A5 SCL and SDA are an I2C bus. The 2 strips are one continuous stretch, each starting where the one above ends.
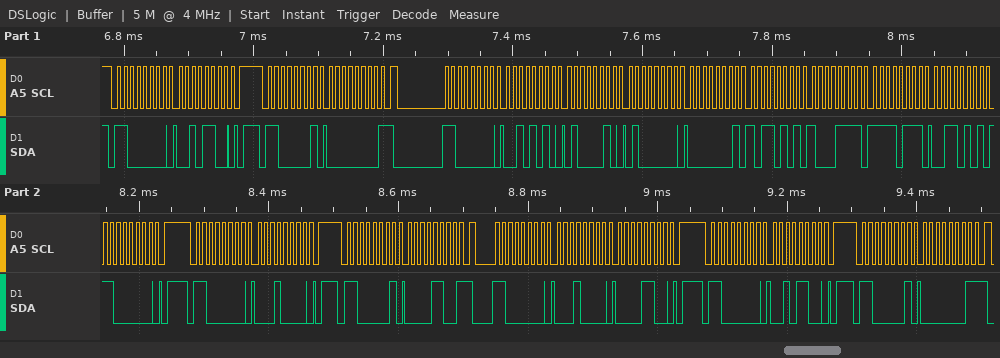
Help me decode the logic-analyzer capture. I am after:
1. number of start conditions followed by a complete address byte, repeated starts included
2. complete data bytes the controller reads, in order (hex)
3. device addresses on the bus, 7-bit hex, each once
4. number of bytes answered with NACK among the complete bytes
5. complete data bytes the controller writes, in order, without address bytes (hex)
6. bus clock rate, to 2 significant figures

8
00 0C 01
0x60
3
2C 2A 42 40 01 B5 8F F7 35 C0 10 10 0C 2C
100 kHz
